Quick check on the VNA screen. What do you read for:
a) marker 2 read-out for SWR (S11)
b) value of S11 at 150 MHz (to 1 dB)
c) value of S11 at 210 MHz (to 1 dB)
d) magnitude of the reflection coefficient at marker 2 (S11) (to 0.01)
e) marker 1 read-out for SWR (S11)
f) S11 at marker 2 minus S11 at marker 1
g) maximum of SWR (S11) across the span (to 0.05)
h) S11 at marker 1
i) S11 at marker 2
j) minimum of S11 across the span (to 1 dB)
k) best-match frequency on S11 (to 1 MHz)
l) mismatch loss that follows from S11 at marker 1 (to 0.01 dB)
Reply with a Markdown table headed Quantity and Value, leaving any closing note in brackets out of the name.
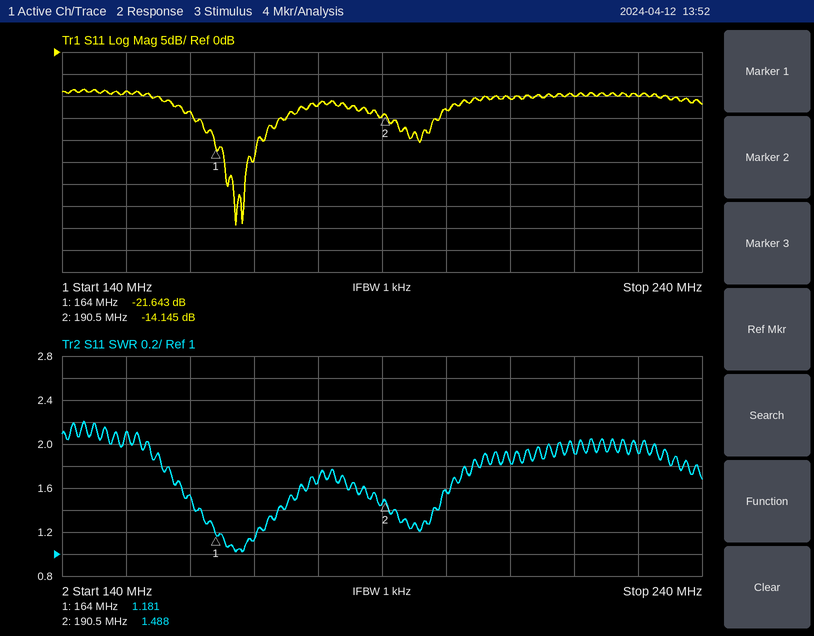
| Quantity | Value |
|---|---|
| marker 2 read-out for SWR | 1.488 |
| value of S11 at 150 MHz | -9 dB |
| value of S11 at 210 MHz | -11 dB |
| magnitude of the reflection coefficient at marker 2 (S11) | 0.20 |
| marker 1 read-out for SWR | 1.181 |
| S11 at marker 2 minus S11 at marker 1 | 7.498 dB |
| maximum of SWR (S11) across the span | 2.20 |
| S11 at marker 1 | -21.643 dB |
| S11 at marker 2 | -14.145 dB |
| minimum of S11 across the span | -39 dB |
| best-match frequency on S11 | 167 MHz |
| mismatch loss that follows from S11 at marker 1 | 0.03 dB |
